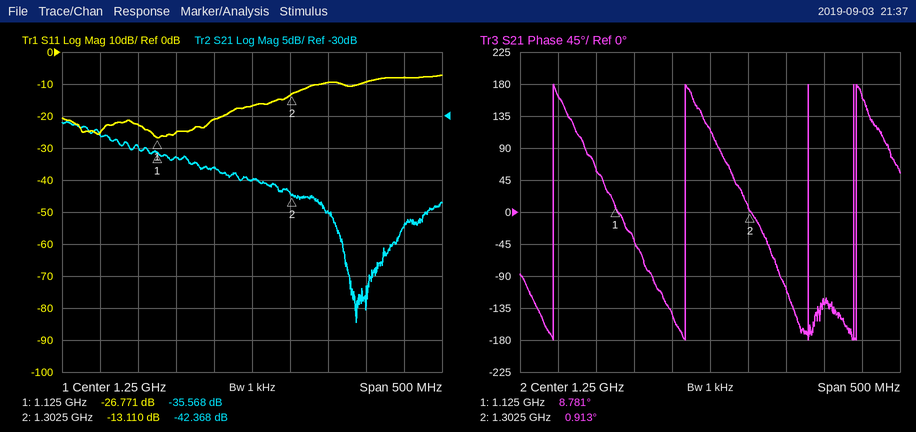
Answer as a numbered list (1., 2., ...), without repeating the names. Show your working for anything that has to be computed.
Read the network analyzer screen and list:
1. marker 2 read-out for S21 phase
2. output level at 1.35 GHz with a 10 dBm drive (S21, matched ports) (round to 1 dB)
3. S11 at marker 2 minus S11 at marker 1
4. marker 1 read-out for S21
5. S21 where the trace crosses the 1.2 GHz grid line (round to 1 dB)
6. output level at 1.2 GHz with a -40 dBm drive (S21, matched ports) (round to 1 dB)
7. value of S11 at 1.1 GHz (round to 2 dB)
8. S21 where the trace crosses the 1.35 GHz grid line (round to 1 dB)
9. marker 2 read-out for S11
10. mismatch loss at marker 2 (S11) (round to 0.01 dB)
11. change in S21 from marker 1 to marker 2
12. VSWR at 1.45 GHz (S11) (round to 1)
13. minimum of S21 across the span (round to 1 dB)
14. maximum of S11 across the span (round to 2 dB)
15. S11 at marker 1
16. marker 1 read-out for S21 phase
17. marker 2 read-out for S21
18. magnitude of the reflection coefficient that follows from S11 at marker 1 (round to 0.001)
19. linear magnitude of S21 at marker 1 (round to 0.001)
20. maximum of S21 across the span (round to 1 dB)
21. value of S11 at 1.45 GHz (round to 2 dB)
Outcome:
1. 0.913°
2. 10 dBm + (-45 dB) = -35 dBm
3. -13.11 − (-26.771) = 13.661 dB
4. -35.568 dB
5. -38 dB
6. -40 dBm + (-38 dB) = -78 dBm
7. -22 dB
8. -45 dB
9. -13.110 dB
10. −10 log10(1 − 10^(-13.11/10)) ≈ 0.22 dB
11. -42.368 − (-35.568) = -6.800 dB
12. |Γ| = 10^(-8/20) = 0.3981; VSWR = (1 + 0.3981)/(1 − 0.3981) ≈ 2
13. -62 dB
14. -8 dB
15. -26.771 dB
16. 8.781°
17. -42.368 dB
18. 10^(-26.771/20) ≈ 0.046
19. 10^(-35.568/20) ≈ 0.017
20. -31 dB
21. -8 dB
